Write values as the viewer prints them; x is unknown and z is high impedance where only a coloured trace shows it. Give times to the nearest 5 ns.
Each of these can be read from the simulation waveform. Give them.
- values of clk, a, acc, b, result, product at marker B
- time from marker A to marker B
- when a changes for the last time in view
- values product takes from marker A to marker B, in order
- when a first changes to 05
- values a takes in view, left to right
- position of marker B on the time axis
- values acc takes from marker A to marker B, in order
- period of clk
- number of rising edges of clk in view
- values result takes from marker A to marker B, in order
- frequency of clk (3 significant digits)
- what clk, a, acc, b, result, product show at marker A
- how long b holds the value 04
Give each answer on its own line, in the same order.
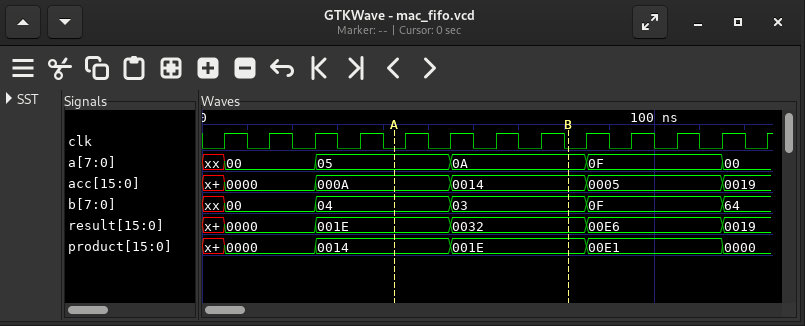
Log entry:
clk=0, a=0A, acc=0014, b=03, result=0032, product=001E
40 ns
115 ns
0014, 001E
25 ns
xx, 00, 05, 0A, 0F, 00
80 ns
000A, 0014
10 ns
13
001E, 0032
100 MHz
clk=0, a=05, acc=000A, b=04, result=001E, product=0014
30 ns
